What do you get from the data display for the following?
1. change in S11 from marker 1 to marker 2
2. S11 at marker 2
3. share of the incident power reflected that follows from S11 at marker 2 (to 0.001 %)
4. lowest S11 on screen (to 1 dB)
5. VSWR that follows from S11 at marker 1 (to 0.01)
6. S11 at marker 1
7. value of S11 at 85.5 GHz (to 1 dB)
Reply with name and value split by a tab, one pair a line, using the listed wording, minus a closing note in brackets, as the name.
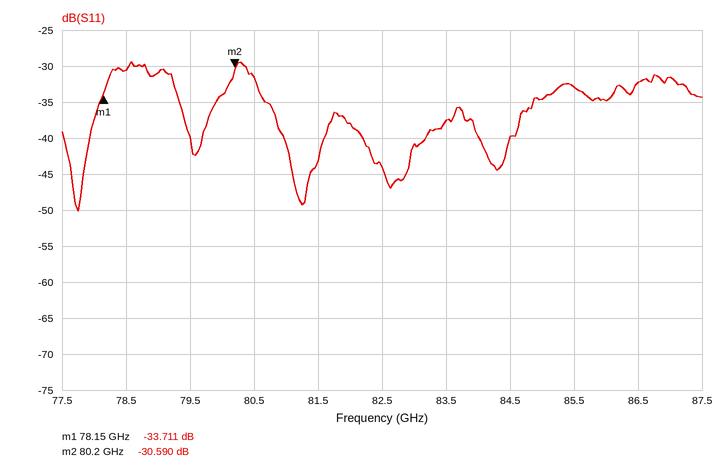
change in S11 from marker 1 to marker 2	3.121 dB
S11 at marker 2	-30.590 dB
share of the incident power reflected that follows from S11 at marker 2	0.087 %
lowest S11 on screen	-50 dB
VSWR that follows from S11 at marker 1	1.04
S11 at marker 1	-33.711 dB
value of S11 at 85.5 GHz	-33 dB
